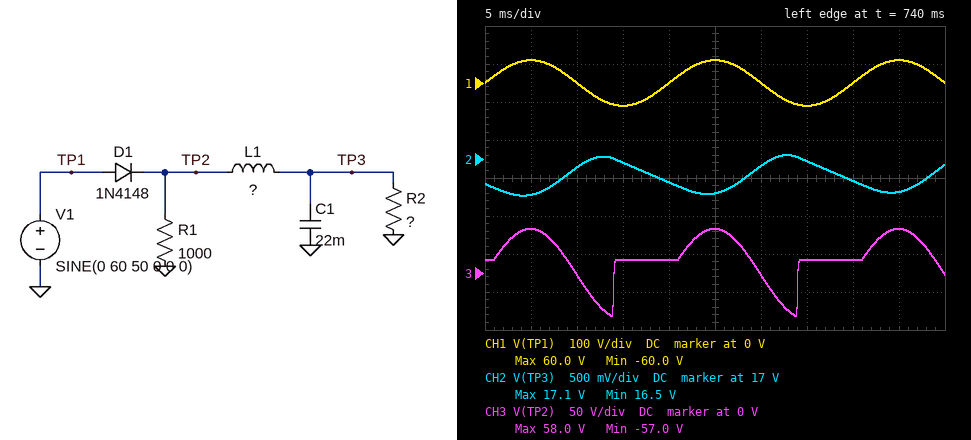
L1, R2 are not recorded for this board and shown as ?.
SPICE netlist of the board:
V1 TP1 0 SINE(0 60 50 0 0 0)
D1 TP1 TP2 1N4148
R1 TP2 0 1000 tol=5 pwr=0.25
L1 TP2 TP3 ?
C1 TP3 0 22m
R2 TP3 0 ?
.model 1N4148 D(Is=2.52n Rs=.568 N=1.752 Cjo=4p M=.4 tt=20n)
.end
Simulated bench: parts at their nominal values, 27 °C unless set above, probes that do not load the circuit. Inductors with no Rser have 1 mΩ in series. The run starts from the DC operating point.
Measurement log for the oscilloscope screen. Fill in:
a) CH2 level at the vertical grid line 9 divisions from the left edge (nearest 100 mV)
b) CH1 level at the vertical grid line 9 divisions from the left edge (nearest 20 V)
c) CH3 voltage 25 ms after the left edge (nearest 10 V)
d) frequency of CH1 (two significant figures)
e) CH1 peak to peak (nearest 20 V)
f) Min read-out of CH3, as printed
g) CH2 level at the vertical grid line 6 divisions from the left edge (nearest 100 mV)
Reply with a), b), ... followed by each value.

a) 16.6 V
b) 60 V
c) 60 V
d) 50 Hz
e) 120 V
f) -57.0 V
g) 16.9 V
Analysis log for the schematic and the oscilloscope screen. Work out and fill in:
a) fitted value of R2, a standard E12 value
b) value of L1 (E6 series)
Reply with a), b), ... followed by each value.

a) 15 Ω
b) 68 mH
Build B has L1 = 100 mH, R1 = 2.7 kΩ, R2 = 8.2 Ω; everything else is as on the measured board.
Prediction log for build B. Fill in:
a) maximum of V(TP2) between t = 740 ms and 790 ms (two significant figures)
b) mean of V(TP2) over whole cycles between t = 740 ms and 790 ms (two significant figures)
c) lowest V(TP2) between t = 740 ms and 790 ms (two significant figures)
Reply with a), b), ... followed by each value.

a) 58 V
b) 9.4 V
c) -61 V
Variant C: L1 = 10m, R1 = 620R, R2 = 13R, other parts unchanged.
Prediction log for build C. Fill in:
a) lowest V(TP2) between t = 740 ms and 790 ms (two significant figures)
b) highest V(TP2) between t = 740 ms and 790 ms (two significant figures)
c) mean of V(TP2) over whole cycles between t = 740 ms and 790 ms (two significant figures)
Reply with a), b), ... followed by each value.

a) -22 V
b) 56 V
c) 32 V
